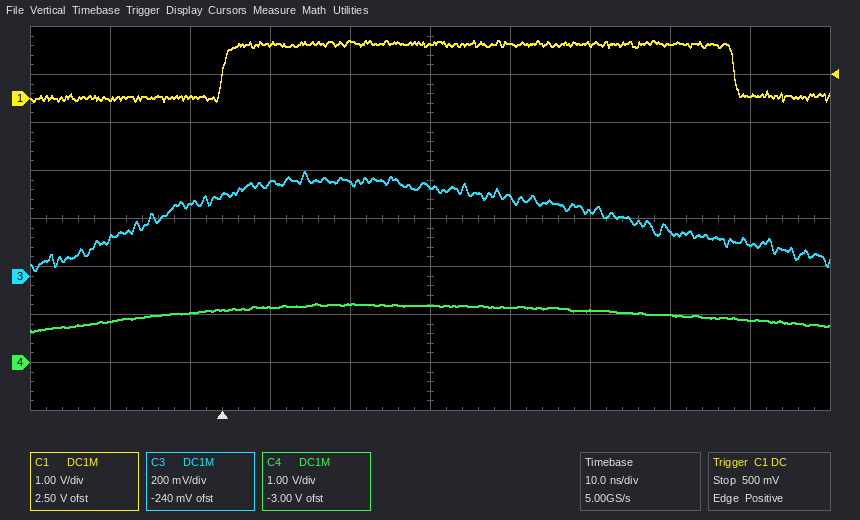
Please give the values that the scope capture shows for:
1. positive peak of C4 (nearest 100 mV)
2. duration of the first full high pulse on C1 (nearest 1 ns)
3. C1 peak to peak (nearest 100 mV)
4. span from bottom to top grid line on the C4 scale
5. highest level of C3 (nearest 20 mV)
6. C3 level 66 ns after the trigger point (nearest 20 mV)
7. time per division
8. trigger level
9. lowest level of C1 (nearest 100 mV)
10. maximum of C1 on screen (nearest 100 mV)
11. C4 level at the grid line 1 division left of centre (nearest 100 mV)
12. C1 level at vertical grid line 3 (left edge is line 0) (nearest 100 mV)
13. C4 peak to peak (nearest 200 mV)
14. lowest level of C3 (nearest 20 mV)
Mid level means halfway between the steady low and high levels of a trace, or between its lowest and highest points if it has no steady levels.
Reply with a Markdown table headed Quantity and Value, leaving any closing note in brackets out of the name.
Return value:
| Quantity | Value |
|---|---|
| positive peak of C4 | 1.2 V |
| duration of the first full high pulse on C1 | 64 ns |
| C1 peak to peak | 1.3 V |
| span from bottom to top grid line on the C4 scale | 8 V |
| highest level of C3 | 440 mV |
| C3 level 66 ns after the trigger point | 140 mV |
| time per division | 10 ns |
| trigger level | 500 mV |
| lowest level of C1 | -100 mV |
| maximum of C1 on screen | 1.2 V |
| C4 level at the grid line 1 division left of centre | 1.2 V |
| C1 level at vertical grid line 3 (left edge is line 0) | 1.1 V |
| C4 peak to peak | 600 mV |
| lowest level of C3 | 20 mV |
